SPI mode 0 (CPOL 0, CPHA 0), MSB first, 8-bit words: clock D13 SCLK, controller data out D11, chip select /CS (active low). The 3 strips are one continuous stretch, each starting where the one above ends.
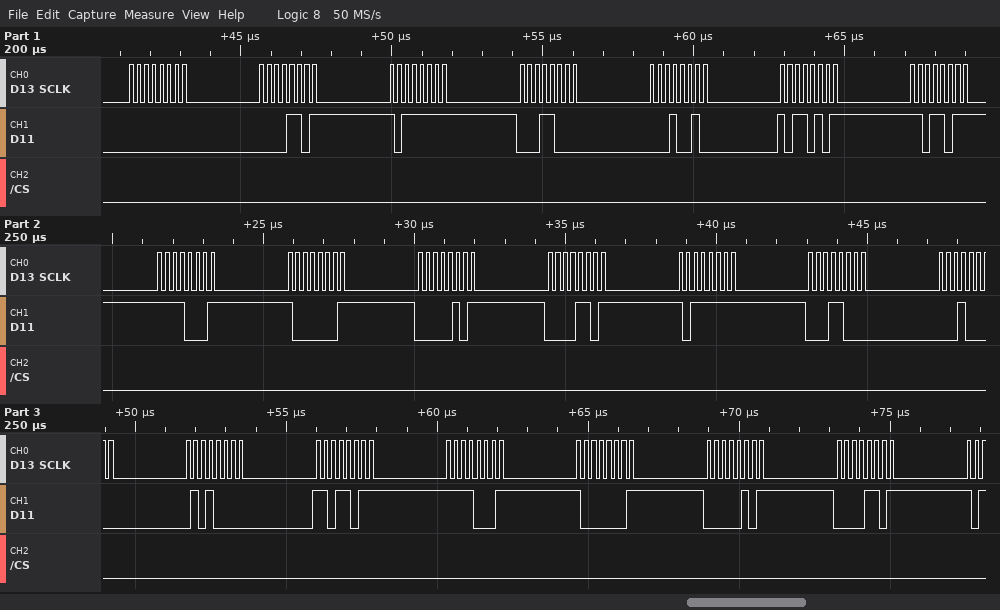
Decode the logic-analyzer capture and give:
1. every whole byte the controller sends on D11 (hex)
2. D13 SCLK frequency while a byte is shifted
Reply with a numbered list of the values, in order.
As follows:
1. 0x00 0x0D 0xBF 0x18 0x12 0xB5 0xDB 0xF1 0x81 0x05 0x0D 0xBF 0x18 0x10 0x50 0xDB 0xF1 0x81 0x05 0x0D
2. 4 MHz
